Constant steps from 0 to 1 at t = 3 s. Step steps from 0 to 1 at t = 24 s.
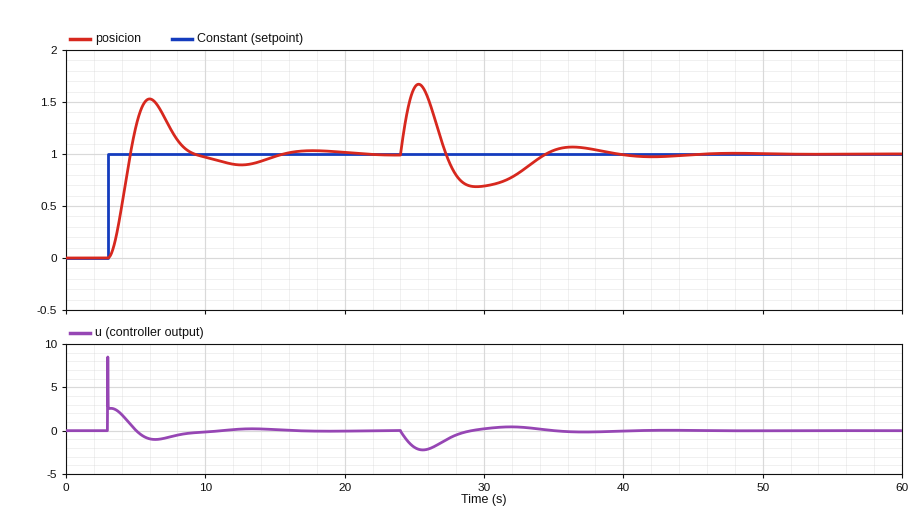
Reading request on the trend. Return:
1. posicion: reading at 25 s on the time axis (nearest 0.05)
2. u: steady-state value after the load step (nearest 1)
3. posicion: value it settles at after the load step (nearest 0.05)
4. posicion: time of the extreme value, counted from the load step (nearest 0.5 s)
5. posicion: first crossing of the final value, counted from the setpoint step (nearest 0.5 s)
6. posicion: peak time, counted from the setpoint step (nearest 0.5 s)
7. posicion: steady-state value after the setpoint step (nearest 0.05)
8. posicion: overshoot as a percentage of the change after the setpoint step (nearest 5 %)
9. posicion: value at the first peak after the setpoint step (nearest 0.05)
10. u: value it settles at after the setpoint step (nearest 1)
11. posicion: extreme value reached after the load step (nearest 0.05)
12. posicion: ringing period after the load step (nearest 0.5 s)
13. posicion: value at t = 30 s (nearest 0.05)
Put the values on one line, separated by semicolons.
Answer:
1.65; 0; 1.00; 1.5 s; 1.5 s; 3.0 s; 1.00; 55 %; 1.55; 0; 1.65; 11.0 s; 0.70
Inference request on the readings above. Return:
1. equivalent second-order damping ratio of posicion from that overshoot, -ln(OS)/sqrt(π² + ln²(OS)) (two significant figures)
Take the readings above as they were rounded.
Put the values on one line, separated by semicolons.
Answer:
0.19
